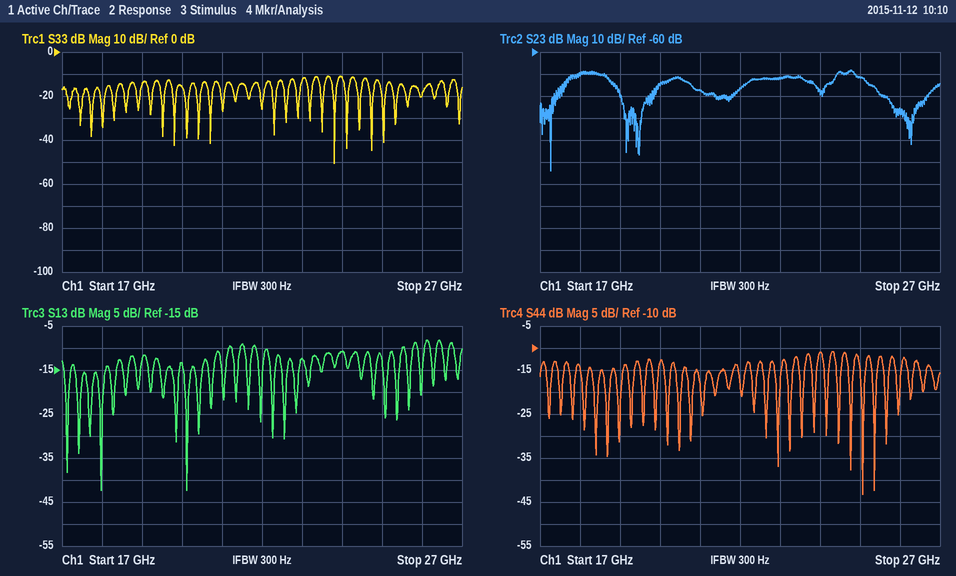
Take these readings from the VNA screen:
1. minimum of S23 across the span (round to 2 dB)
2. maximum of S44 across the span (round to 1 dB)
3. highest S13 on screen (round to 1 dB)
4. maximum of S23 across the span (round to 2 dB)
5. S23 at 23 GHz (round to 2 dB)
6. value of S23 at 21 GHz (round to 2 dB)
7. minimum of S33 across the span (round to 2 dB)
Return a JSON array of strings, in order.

["-114 dB", "-11 dB", "-8 dB", "-68 dB", "-72 dB", "-78 dB", "-50 dB"]
